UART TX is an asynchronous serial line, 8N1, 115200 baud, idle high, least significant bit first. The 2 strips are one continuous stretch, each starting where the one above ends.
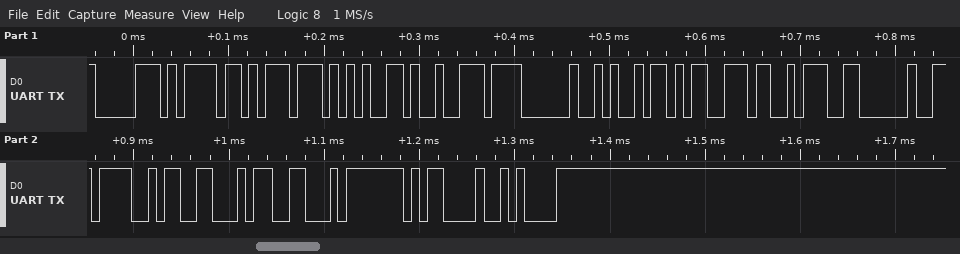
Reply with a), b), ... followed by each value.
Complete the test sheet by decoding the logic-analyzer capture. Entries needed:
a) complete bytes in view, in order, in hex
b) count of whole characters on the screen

a) 0x70 0x6F 0x77 0x65 0x72 0x20 0x69 0x73 0x3A 0x20 0x4F 0x46 0x46 0x0D 0x0A
b) 15
